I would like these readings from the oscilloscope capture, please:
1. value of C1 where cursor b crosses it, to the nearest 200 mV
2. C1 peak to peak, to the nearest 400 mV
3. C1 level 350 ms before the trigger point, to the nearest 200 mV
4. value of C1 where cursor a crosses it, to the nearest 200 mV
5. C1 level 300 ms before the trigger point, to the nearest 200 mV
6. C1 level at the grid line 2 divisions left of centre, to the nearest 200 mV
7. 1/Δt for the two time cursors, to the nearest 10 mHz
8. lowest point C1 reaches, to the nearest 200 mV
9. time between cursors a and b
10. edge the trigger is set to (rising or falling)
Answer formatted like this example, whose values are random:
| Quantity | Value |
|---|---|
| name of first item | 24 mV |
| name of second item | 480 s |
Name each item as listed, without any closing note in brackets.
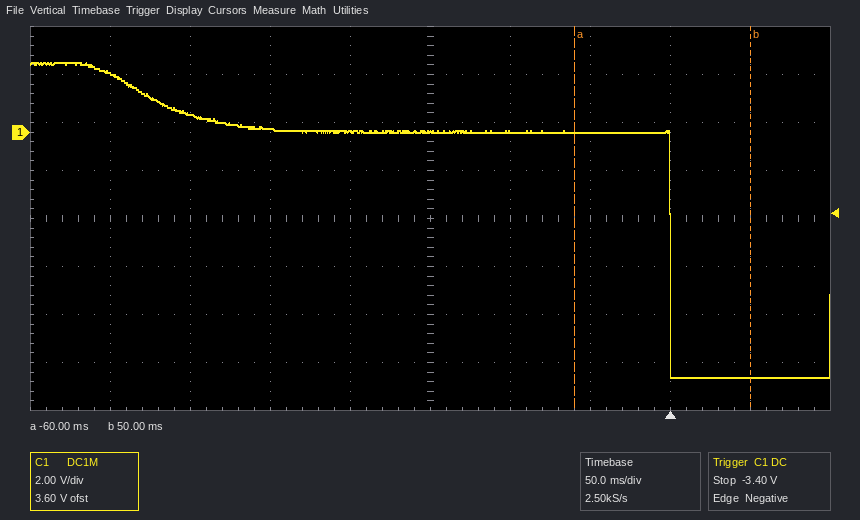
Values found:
| Quantity | Value |
|---|---|
| value of C1 where cursor b crosses it, to the nearest 200 mV | -10.2 V |
| C1 peak to peak, to the nearest 400 mV | 13.2 V |
| C1 level 350 ms before the trigger point, to the nearest 200 mV | 2.4 V |
| value of C1 where cursor a crosses it, to the nearest 200 mV | 0.0 V |
| C1 level 300 ms before the trigger point, to the nearest 200 mV | 800 mV |
| C1 level at the grid line 2 divisions left of centre, to the nearest 200 mV | 200 mV |
| 1/Δt for the two time cursors, to the nearest 10 mHz | 9.09 Hz |
| lowest point C1 reaches, to the nearest 200 mV | -10.2 V |
| time between cursors a and b | 110 ms |
| edge the trigger is set to | falling |
